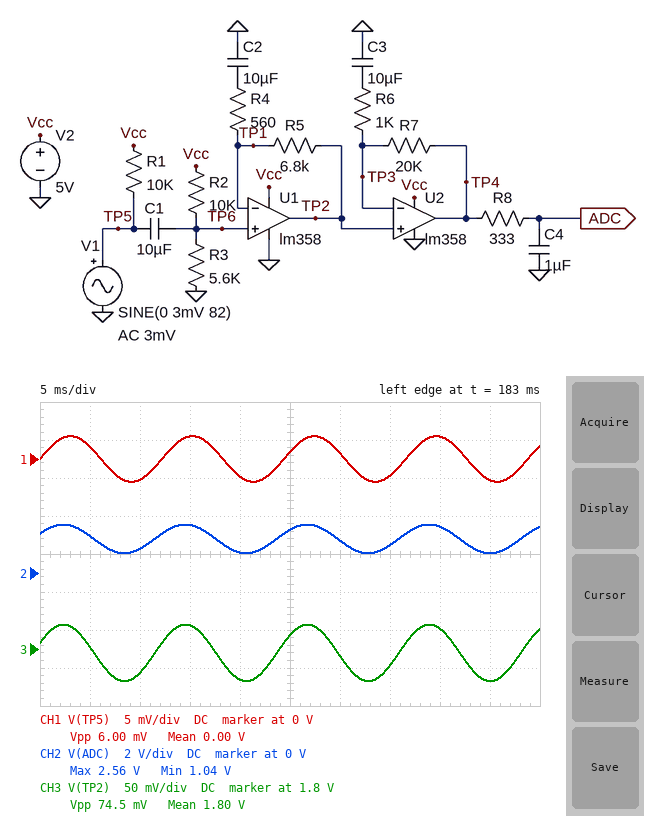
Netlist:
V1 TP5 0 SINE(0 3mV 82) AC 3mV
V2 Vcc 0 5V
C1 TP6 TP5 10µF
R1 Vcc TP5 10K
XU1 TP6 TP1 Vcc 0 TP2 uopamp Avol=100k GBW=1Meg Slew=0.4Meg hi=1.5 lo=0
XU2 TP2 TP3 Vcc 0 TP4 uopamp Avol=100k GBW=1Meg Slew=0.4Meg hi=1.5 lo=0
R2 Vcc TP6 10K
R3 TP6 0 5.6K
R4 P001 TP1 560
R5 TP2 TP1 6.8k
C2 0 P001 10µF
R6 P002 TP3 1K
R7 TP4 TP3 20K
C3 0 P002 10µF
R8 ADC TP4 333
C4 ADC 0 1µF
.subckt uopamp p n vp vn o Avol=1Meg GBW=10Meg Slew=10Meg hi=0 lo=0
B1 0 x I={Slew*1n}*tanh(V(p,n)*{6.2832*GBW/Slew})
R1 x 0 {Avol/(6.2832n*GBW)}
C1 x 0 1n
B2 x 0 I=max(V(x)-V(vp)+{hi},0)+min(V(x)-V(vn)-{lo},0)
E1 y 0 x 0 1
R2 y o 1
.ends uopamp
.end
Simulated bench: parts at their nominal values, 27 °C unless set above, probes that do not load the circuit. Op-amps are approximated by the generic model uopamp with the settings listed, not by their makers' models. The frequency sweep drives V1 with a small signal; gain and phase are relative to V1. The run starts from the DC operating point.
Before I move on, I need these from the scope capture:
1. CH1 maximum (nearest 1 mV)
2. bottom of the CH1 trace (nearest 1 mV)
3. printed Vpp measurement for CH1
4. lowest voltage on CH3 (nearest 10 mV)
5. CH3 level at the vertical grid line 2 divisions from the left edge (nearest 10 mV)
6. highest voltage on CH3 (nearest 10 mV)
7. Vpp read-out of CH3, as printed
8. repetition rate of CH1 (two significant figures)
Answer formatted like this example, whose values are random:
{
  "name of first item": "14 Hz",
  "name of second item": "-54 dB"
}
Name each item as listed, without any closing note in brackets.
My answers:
{
  "CH1 maximum": "3 mV",
  "bottom of the CH1 trace": "-3 mV",
  "printed Vpp measurement for CH1": "6.00 mV",
  "lowest voltage on CH3": "1.76 V",
  "CH3 level at the vertical grid line 2 divisions from the left edge": "1.77 V",
  "highest voltage on CH3": "1.83 V",
  "Vpp read-out of CH3, as printed": "74.5 mV",
  "repetition rate of CH1": "82 Hz"
}
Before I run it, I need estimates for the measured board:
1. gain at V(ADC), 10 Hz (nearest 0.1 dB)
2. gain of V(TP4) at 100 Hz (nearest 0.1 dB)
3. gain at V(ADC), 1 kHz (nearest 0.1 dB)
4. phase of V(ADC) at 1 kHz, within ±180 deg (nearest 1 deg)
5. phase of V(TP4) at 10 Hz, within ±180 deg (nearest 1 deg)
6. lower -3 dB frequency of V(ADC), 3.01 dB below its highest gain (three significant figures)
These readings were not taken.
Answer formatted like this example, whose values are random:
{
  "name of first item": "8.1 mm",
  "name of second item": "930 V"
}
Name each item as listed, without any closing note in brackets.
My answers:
{
  "gain at V(ADC), 10 Hz": "33.2 dB",
  "gain of V(TP4) at 100 Hz": "48.4 dB",
  "gain at V(ADC), 1 kHz": "41.5 dB",
  "phase of V(ADC) at 1 kHz, within ±180 deg": "-64 deg",
  "phase of V(TP4) at 10 Hz, within ±180 deg": "136 deg",
  "lower -3 dB frequency of V(ADC), 3.01 dB below its highest gain": "31.9 Hz"
}
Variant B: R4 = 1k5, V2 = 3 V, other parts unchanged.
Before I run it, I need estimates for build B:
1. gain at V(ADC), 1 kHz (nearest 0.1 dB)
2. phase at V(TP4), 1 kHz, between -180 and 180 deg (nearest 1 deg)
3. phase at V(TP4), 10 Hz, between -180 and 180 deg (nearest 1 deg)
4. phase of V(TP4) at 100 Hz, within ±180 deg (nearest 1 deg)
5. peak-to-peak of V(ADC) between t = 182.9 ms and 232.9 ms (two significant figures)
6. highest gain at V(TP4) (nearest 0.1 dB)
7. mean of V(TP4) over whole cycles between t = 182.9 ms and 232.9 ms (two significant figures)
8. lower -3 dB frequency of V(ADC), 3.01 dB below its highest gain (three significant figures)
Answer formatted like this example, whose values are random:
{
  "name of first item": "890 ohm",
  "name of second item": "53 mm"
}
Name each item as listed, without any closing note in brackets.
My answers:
{
  "gain at V(ADC), 1 kHz": "34.0 dB",
  "phase at V(TP4), 1 kHz, between -180 and 180 deg": "0 deg",
  "phase at V(TP4), 10 Hz, between -180 and 180 deg": "113 deg",
  "phase of V(TP4) at 100 Hz, within ±180 deg": "16 deg",
  "peak-to-peak of V(ADC) between t = 182.9 ms and 232.9 ms": "670 mV",
  "highest gain at V(TP4)": "41.3 dB",
  "mean of V(TP4) over whole cycles between t = 182.9 ms and 232.9 ms": "1.1 V",
  "lower -3 dB frequency of V(ADC), 3.01 dB below its highest gain": "20.1 Hz"
}
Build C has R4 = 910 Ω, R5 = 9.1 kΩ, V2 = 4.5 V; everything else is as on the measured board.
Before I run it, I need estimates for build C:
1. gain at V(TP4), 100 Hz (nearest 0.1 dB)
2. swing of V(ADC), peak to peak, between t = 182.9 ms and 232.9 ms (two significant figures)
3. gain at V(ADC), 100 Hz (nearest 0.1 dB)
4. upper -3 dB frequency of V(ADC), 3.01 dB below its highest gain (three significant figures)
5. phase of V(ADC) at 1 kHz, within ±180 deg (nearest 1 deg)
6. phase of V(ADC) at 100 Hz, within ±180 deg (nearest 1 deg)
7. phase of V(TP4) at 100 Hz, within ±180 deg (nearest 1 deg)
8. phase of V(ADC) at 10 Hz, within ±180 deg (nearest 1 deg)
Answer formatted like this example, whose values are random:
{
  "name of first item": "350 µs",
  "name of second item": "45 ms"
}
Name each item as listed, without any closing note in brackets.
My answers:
{
  "gain at V(TP4), 100 Hz": "47.0 dB",
  "swing of V(ADC), peak to peak, between t = 182.9 ms and 232.9 ms": "1.3 V",
  "gain at V(ADC), 100 Hz": "46.8 dB",
  "upper -3 dB frequency of V(ADC), 3.01 dB below its highest gain": "524 Hz",
  "phase of V(ADC) at 1 kHz, within ±180 deg": "-64 deg",
  "phase of V(ADC) at 100 Hz, within ±180 deg": "8 deg",
  "phase of V(TP4) at 100 Hz, within ±180 deg": "20 deg",
  "phase of V(ADC) at 10 Hz, within ±180 deg": "127 deg"
}
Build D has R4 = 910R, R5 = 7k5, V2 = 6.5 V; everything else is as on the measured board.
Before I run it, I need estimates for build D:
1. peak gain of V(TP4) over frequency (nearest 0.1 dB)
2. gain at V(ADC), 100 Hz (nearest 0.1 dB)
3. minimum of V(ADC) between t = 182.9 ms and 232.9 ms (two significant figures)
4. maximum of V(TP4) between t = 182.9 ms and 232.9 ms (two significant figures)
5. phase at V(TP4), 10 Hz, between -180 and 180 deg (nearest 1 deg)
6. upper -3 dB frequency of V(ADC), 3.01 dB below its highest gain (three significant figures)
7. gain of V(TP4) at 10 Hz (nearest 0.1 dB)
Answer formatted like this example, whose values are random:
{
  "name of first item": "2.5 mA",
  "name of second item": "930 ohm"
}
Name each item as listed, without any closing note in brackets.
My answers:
{
  "peak gain of V(TP4) over frequency": "45.8 dB",
  "gain at V(ADC), 100 Hz": "45.3 dB",
  "minimum of V(ADC) between t = 182.9 ms and 232.9 ms": "1.8 V",
  "maximum of V(TP4) between t = 182.9 ms and 232.9 ms": "2.9 V",
  "phase at V(TP4), 10 Hz, between -180 and 180 deg": "127 deg",
  "upper -3 dB frequency of V(ADC), 3.01 dB below its highest gain": "524 Hz",
  "gain of V(TP4) at 10 Hz": "33.6 dB"
}
